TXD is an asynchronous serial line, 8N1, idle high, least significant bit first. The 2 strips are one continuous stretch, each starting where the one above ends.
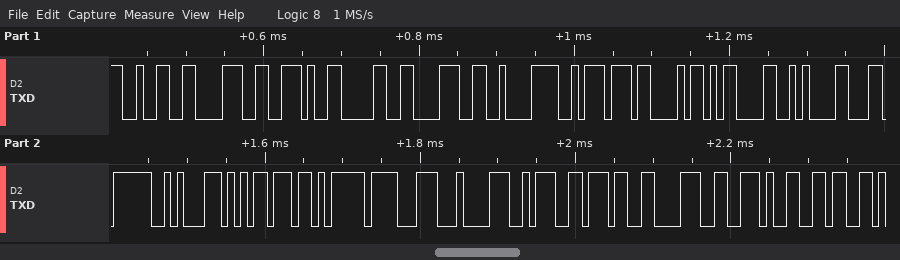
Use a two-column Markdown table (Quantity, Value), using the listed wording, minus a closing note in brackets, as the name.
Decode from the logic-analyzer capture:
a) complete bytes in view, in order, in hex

| Quantity | Value |
|---|---|
| complete bytes in view, in order, in hex | 32 38 2E 30 38 C2 BA 43 0D 0A EC 8A B5 EB 8F 84 3A 37 38 2E 36 |
